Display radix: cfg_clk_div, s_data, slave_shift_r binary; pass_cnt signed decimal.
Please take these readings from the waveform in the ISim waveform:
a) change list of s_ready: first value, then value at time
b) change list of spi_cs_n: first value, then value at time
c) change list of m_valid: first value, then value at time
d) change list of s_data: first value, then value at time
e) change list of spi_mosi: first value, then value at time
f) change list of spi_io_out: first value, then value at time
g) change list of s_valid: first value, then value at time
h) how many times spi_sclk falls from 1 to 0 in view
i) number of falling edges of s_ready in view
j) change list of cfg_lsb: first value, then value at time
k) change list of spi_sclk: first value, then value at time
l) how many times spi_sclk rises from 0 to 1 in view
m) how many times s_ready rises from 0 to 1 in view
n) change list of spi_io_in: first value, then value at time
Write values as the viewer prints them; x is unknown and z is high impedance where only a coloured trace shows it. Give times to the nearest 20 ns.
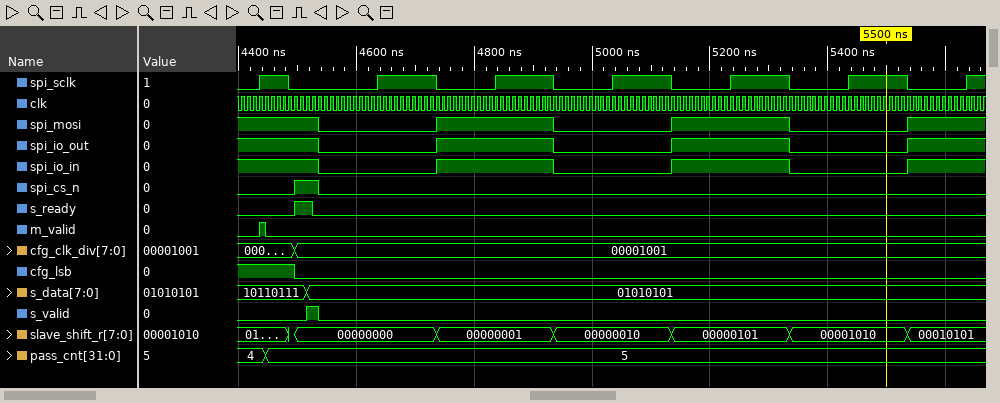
0, 1 at 4500 ns, 0 at 4520 ns
0, 1 at 4500 ns, 0 at 4540 ns
0, 1 at 4440 ns, 0 at 4440 ns
10110111, 01010101 at 4520 ns
1, 0 at 4540 ns, 1 at 4740 ns, 0 at 4940 ns, 1 at 5140 ns, 0 at 5340 ns, 1 at 5540 ns
1, 0 at 4540 ns, 1 at 4740 ns, 0 at 4940 ns, 1 at 5140 ns, 0 at 5340 ns, 1 at 5540 ns
0, 1 at 4520 ns, 0 at 4540 ns
6
1
1, 0 at 4500 ns
0, 1 at 4440 ns, 0 at 4480 ns, 1 at 4640 ns, 0 at 4740 ns, 1 at 4840 ns, 0 at 4940 ns, 1 at 5040 ns, 0 at 5140 ns, 1 at 5240 ns, 0 at 5340 ns, 1 at 5440 ns, 0 at 5540 ns, 1 at 5640 ns
7
1
1, 0 at 4540 ns, 1 at 4740 ns, 0 at 4940 ns, 1 at 5140 ns, 0 at 5340 ns, 1 at 5540 ns
